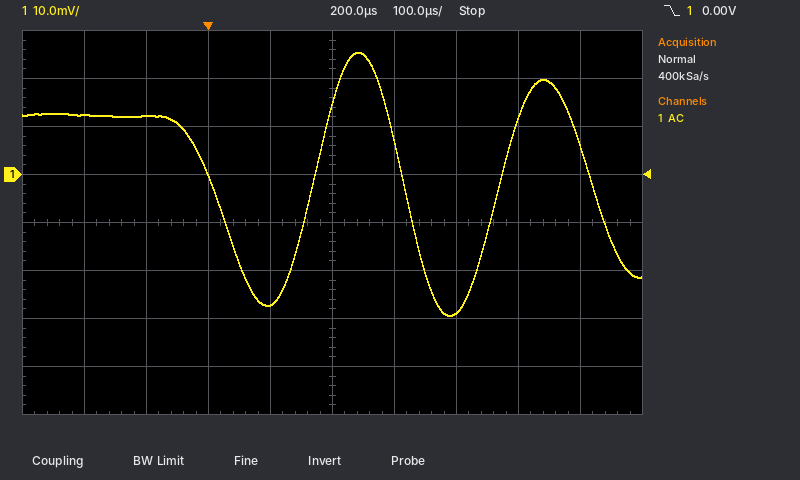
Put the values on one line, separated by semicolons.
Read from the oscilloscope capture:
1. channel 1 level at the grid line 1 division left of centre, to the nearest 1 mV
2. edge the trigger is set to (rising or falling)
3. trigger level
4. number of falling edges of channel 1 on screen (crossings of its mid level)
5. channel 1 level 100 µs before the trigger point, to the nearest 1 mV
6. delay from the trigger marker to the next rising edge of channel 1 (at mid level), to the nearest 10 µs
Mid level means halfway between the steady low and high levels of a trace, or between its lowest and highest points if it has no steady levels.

-27 mV; falling; 0.00 V; 3; 12 mV; 170 µs
